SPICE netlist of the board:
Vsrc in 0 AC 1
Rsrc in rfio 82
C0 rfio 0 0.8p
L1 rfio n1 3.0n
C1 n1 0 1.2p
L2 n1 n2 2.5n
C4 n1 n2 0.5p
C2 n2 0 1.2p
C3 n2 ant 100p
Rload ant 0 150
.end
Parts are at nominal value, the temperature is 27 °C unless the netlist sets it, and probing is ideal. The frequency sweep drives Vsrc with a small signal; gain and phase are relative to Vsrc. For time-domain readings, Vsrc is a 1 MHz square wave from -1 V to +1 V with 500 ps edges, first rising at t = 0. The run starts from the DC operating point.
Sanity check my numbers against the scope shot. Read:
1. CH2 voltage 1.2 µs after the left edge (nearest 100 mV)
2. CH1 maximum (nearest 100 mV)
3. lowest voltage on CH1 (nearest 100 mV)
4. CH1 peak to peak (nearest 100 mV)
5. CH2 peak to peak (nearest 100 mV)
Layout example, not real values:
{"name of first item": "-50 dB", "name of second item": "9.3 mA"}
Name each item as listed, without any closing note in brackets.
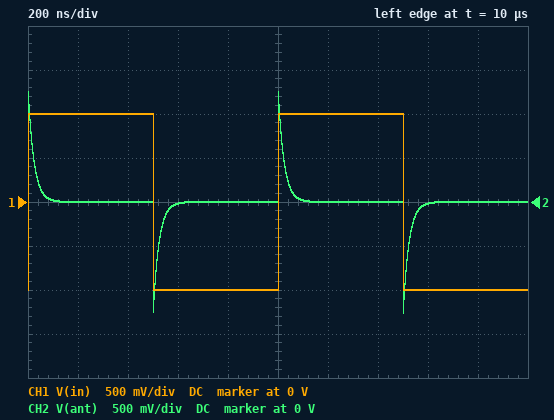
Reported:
{"CH2 voltage 1.2 µs after the left edge": "0 V", "CH1 maximum": "1.0 V", "lowest voltage on CH1": "-1.0 V", "CH1 peak to peak": "2.0 V", "CH2 peak to peak": "2.5 V"}
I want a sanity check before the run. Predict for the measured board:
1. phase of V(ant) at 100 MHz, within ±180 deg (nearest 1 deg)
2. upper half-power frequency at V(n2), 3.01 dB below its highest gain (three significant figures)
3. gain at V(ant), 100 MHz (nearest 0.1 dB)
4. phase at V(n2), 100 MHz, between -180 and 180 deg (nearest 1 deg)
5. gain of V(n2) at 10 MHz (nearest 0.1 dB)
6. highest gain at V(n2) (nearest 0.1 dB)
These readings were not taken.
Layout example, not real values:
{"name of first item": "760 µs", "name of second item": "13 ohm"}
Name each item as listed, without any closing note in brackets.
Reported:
{"phase of V(ant) at 100 MHz, within ±180 deg": "-3 deg", "upper half-power frequency at V(n2), 3.01 dB below its highest gain": "16.6 MHz", "gain at V(ant), 100 MHz": "-3.9 dB", "phase at V(n2), 100 MHz, between -180 and 180 deg": "-9 deg", "gain of V(n2) at 10 MHz": "-2.2 dB", "highest gain at V(n2)": "0 dB"}
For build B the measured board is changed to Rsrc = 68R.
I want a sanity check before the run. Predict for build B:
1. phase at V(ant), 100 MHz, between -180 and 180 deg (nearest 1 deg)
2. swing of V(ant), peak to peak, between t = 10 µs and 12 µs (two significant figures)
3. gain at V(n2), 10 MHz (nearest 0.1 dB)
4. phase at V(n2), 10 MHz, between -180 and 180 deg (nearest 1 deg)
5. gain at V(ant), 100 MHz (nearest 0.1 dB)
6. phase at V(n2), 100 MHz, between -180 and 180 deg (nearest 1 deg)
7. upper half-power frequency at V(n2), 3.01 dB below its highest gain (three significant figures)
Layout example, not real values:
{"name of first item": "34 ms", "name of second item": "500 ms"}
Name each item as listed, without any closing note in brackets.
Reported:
{"phase at V(ant), 100 MHz, between -180 and 180 deg": "-2 deg", "swing of V(ant), peak to peak, between t = 10 µs and 12 µs": "2.7 V", "gain at V(n2), 10 MHz": "-1.8 dB", "phase at V(n2), 10 MHz, between -180 and 180 deg": "-11 deg", "gain at V(ant), 100 MHz": "-3.3 dB", "phase at V(n2), 100 MHz, between -180 and 180 deg": "-8 deg", "upper half-power frequency at V(n2), 3.01 dB below its highest gain": "30.4 MHz"}
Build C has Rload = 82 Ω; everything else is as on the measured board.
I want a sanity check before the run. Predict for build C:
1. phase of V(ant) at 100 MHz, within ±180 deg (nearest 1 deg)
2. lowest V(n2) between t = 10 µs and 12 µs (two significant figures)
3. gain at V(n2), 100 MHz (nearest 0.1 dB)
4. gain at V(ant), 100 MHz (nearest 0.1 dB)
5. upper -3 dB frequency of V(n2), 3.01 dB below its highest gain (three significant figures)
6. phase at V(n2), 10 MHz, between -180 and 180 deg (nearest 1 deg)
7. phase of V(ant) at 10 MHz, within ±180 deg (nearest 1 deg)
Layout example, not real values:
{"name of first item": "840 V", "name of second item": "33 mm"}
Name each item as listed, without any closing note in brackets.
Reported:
{"phase of V(ant) at 100 MHz, within ±180 deg": "0 deg", "lowest V(n2) between t = 10 µs and 12 µs": "-1.0 V", "gain at V(n2), 100 MHz": "-6.0 dB", "gain at V(ant), 100 MHz": "-6.1 dB", "upper -3 dB frequency of V(n2), 3.01 dB below its highest gain": "13.6 MHz", "phase at V(n2), 10 MHz, between -180 and 180 deg": "-19 deg", "phase of V(ant) at 10 MHz, within ±180 deg": "43 deg"}
